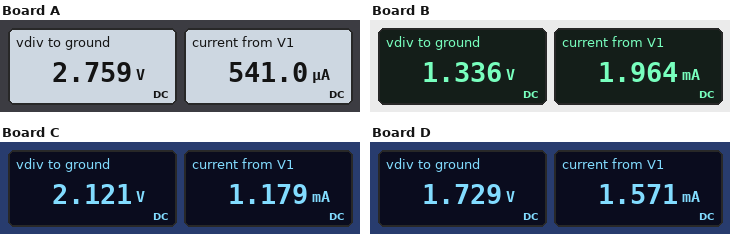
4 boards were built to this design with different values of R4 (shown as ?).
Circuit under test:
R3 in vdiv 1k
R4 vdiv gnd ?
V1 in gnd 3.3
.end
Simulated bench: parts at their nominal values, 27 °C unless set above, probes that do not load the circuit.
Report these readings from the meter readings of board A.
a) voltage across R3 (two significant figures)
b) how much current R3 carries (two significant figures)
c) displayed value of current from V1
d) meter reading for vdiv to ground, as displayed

540 mV
540 µA
541.0 µA
2.759 V
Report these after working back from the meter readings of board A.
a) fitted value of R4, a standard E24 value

5.1 kΩ
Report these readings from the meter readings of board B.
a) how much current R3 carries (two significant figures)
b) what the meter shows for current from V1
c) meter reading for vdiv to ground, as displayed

2.0 mA
1.964 mA
1.336 V
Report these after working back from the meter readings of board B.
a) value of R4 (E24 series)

680 Ω
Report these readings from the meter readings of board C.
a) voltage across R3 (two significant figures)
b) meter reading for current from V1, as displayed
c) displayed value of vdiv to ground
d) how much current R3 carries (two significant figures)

1.2 V
1.179 mA
2.121 V
1.2 mA
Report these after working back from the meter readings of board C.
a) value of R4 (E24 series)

1.8 kΩ
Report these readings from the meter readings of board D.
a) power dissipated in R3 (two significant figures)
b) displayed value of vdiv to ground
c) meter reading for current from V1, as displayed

2.5 mW
1.729 V
1.571 mA
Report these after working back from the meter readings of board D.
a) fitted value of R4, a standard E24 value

1.1 kΩ
